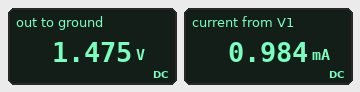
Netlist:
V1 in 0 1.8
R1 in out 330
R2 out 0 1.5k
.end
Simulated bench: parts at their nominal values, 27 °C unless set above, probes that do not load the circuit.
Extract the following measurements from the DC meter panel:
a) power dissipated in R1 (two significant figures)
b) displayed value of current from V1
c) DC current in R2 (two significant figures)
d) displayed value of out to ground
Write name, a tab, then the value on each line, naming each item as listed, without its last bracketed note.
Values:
power dissipated in R1	320 µW
displayed value of current from V1	0.984 mA
DC current in R2	980 µA
displayed value of out to ground	1.475 V
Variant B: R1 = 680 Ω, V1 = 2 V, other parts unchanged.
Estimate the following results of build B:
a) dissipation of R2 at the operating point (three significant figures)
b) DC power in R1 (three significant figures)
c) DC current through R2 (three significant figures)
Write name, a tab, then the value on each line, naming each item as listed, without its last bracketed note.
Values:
dissipation of R2 at the operating point	1.26 mW
DC power in R1	572 µW
DC current through R2	917 µA
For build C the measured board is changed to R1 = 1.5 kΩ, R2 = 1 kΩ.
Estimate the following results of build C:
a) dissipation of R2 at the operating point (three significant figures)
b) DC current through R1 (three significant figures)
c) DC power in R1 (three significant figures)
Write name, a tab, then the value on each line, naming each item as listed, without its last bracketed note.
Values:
dissipation of R2 at the operating point	518 µW
DC current through R1	720 µA
DC power in R1	778 µW
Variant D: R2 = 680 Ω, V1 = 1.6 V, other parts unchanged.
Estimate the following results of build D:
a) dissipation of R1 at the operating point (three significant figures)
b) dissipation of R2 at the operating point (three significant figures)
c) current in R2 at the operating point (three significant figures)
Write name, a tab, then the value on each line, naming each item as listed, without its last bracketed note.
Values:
dissipation of R1 at the operating point	828 µW
dissipation of R2 at the operating point	1.71 mW
current in R2 at the operating point	1.58 mA
